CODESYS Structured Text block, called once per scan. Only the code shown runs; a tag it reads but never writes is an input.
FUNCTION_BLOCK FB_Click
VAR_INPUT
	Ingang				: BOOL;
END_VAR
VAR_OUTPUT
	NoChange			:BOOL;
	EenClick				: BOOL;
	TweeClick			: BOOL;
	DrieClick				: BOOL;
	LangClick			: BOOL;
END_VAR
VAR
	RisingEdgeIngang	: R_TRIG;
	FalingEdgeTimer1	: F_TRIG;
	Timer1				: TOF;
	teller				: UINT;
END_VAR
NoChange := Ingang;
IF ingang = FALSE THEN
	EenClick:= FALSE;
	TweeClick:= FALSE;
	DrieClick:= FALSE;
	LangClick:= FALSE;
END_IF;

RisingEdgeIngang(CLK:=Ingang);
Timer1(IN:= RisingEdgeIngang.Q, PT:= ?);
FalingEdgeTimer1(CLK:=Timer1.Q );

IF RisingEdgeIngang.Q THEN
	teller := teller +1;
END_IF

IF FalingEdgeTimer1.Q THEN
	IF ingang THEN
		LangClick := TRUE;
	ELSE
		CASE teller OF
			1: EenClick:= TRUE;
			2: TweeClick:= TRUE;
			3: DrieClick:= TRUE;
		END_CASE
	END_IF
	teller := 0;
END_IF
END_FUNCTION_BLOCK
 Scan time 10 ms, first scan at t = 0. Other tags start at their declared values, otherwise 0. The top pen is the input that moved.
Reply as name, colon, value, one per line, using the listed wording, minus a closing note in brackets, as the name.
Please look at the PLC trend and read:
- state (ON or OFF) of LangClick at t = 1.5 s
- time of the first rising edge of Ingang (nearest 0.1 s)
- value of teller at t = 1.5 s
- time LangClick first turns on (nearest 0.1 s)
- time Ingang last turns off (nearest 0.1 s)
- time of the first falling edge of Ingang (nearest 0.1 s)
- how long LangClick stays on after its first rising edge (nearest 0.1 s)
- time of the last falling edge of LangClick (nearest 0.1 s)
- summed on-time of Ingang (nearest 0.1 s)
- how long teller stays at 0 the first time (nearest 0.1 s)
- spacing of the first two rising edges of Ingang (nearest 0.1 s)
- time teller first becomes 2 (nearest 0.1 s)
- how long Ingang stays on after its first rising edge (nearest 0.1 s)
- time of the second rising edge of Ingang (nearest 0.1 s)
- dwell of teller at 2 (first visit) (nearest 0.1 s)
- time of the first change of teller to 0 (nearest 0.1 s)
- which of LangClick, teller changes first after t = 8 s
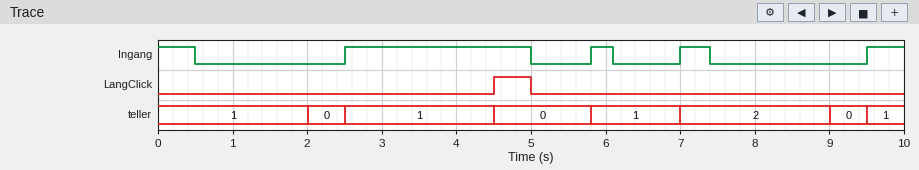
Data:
state (ON or OFF) of LangClick at t = 1.5 s: OFF
time of the first rising edge of Ingang: 2.5 s
value of teller at t = 1.5 s: 1
time LangClick first turns on: 4.5 s
time Ingang last turns off: 7.4 s
time of the first falling edge of Ingang: 0.5 s
how long LangClick stays on after its first rising edge: 0.5 s
time of the last falling edge of LangClick: 5.0 s
summed on-time of Ingang: 4.2 s
how long teller stays at 0 the first time: 0.5 s
spacing of the first two rising edges of Ingang: 3.3 s
time teller first becomes 2: 7.0 s
how long Ingang stays on after its first rising edge: 2.5 s
time of the second rising edge of Ingang: 5.8 s
dwell of teller at 2 (first visit): 2.0 s
time of the first change of teller to 0: 2.0 s
which of LangClick, teller changes first after t = 8 s: teller
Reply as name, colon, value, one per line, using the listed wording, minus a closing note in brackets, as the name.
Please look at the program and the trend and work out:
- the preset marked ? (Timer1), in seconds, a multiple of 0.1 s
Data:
the preset marked ? (Timer1), in seconds, a multiple of 0.1 s: 2.0 s
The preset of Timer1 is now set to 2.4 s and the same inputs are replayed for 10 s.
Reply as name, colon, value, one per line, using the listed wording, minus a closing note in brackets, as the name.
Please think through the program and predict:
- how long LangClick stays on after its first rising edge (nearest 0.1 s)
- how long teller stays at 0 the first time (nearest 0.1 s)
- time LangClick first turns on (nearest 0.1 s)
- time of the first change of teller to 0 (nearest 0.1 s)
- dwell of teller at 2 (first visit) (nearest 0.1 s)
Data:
how long LangClick stays on after its first rising edge: 0.1 s
how long teller stays at 0 the first time: 0.1 s
time LangClick first turns on: 4.9 s
time of the first change of teller to 0: 2.4 s
dwell of teller at 2 (first visit): 2.4 s
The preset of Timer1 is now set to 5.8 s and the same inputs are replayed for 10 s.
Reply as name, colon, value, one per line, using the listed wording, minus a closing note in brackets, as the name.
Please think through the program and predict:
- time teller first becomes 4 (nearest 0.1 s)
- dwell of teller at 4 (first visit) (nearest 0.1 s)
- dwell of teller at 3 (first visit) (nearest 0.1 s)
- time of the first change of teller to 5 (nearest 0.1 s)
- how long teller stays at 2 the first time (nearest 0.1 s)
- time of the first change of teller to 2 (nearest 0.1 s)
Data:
time teller first becomes 4: 7.0 s
dwell of teller at 4 (first visit): 2.5 s
dwell of teller at 3 (first visit): 1.2 s
time of the first change of teller to 5: 9.5 s
how long teller stays at 2 the first time: 3.3 s
time of the first change of teller to 2: 2.5 s
